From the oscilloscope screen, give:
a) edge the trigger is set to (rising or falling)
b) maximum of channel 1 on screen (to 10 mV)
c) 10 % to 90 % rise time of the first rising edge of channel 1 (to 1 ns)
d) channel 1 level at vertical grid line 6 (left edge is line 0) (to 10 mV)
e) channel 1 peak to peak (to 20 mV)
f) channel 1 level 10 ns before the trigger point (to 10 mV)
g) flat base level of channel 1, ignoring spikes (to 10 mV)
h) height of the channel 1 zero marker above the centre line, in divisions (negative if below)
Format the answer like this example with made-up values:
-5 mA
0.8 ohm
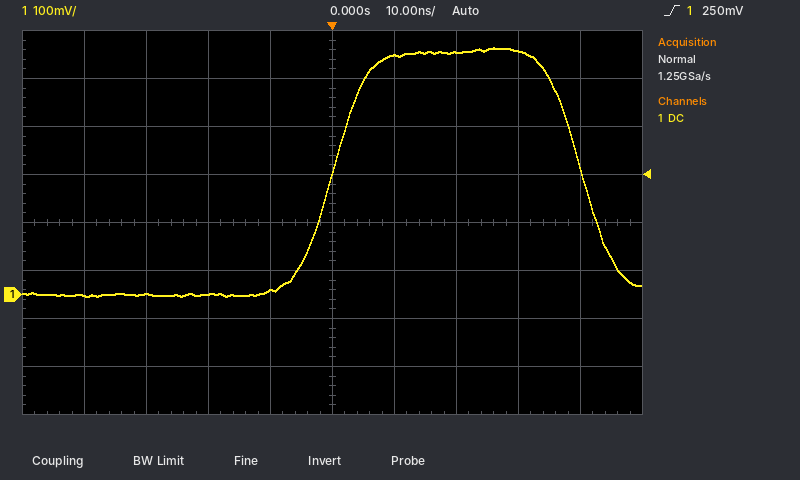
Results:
rising
510 mV
11 ns
500 mV
520 mV
10 mV
0 mV
-1.5 div
